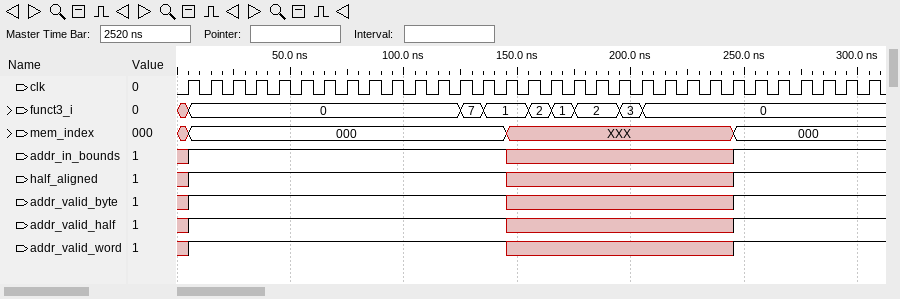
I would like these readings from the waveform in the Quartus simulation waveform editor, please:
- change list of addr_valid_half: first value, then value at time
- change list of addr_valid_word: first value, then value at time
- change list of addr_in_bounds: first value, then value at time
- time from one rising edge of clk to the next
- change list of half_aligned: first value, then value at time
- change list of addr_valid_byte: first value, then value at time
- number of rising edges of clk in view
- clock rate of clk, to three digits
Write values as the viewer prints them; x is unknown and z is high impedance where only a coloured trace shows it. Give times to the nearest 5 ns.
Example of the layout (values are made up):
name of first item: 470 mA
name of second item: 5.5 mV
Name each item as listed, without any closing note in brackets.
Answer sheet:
change list of addr_valid_half: first value, then value at time: x, 1 at 5 ns, x at 145 ns, 1 at 245 ns
change list of addr_valid_word: first value, then value at time: x, 1 at 5 ns, x at 145 ns, 1 at 245 ns
change list of addr_in_bounds: first value, then value at time: x, 1 at 5 ns, x at 145 ns, 1 at 245 ns
time from one rising edge of clk to the next: 10 ns
change list of half_aligned: first value, then value at time: x, 1 at 5 ns, x at 145 ns, 1 at 245 ns
change list of addr_valid_byte: first value, then value at time: x, 1 at 5 ns, x at 145 ns, 1 at 245 ns
number of rising edges of clk in view: 31
clock rate of clk, to three digits: 100 MHz
